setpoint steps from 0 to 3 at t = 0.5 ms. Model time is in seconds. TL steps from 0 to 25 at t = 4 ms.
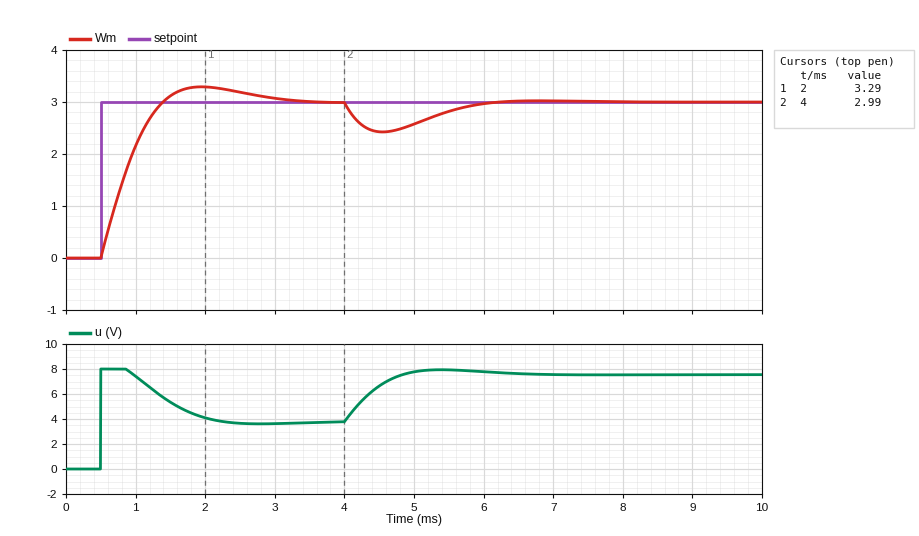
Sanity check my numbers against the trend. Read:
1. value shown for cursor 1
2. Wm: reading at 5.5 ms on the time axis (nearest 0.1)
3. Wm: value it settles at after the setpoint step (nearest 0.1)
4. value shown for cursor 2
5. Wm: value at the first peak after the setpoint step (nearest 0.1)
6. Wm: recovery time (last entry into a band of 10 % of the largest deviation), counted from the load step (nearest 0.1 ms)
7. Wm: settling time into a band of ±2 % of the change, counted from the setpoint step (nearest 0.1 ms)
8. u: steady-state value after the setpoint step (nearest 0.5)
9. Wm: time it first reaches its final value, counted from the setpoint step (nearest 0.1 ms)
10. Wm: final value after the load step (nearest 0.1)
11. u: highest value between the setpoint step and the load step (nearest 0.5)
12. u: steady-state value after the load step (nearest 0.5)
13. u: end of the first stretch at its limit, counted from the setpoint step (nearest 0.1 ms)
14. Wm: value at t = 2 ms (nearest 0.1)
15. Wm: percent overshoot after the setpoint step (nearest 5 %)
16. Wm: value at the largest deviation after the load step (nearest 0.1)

3.29
2.8
3.0
2.99
3.3
1.9 ms
2.6 ms
4.0
0.9 ms
3.0
8.0
7.5
0.4 ms
3.3
10 %
2.4
